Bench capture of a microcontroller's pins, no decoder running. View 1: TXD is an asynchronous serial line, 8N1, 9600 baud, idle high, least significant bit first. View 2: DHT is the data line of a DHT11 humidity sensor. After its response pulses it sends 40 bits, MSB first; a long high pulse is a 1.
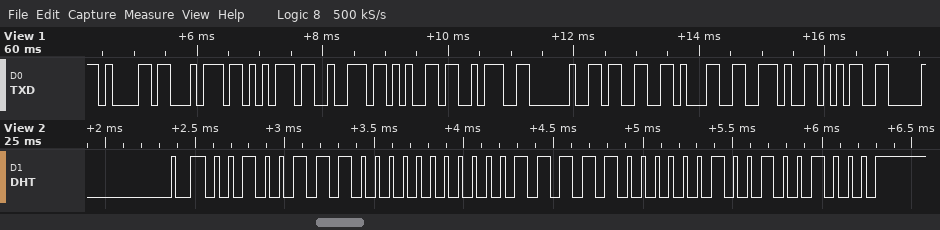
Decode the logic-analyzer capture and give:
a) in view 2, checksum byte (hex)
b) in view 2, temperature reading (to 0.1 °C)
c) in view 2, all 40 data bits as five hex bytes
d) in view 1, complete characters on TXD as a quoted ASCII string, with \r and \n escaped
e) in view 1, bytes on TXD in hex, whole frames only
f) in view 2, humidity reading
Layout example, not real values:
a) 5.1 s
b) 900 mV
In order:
a) 0x48
b) 31.2 °C
c) 27 00 1F 02 48
d) "ature: 31.5"
e) 61 74 75 72 65 3A 20 33 31 2E 35
f) 39 %
